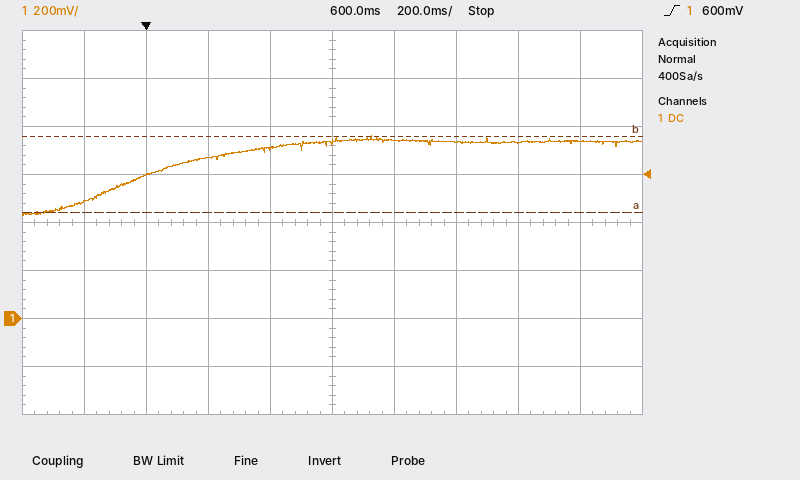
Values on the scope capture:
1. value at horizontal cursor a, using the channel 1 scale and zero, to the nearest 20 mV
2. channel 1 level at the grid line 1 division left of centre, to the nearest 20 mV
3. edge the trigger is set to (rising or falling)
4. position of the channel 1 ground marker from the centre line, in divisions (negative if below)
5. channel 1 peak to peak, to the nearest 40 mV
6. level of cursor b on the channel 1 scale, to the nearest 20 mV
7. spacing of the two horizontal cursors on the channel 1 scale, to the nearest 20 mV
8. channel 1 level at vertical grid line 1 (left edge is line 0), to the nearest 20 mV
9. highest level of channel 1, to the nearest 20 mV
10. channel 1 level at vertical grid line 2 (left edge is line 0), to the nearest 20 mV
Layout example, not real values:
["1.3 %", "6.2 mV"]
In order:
["440 mV", "700 mV", "rising", "-2.0 div", "320 mV", "760 mV", "320 mV", "480 mV", "760 mV", "600 mV"]
